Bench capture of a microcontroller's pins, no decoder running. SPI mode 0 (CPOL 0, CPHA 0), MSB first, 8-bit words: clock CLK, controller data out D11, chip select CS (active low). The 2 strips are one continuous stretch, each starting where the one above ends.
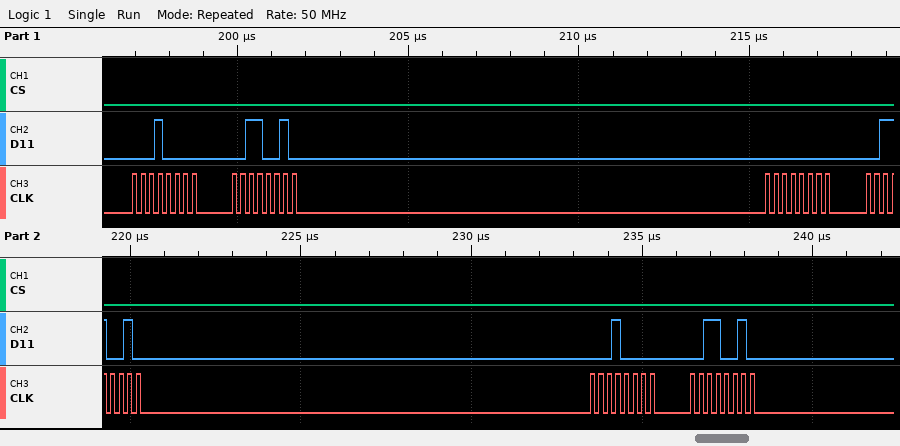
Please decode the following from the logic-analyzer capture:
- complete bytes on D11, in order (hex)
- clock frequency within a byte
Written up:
0x10 0x32 0x00 0x32 0x10 0x32
4 MHz
